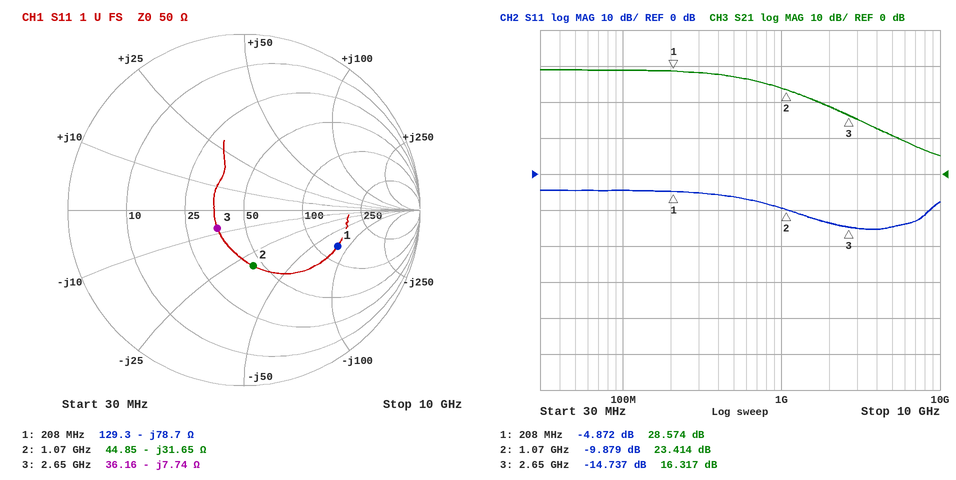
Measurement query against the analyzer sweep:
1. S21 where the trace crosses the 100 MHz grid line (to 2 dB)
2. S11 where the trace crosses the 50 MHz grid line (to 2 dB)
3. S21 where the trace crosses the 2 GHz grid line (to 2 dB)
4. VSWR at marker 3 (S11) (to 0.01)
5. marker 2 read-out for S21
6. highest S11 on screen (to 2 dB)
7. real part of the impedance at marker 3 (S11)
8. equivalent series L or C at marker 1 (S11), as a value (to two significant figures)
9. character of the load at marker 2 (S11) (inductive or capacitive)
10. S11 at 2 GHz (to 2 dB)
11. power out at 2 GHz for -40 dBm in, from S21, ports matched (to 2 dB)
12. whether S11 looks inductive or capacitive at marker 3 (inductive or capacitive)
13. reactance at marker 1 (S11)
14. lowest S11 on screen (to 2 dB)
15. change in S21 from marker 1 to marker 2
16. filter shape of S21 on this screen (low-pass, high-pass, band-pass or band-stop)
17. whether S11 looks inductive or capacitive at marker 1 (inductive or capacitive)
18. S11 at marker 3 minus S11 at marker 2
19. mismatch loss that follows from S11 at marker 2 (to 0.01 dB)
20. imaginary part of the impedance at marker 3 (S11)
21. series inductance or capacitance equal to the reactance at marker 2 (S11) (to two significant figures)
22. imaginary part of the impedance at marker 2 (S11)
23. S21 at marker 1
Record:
28 dB
-4 dB
18 dB
1.45
23.414 dB
-4 dB
36.16 Ω
9.7 pF
capacitive
-14 dB
-22 dBm
capacitive
-78.7 Ω
-16 dB
-5.160 dB
low-pass
capacitive
-4.858 dB
0.47 dB
-7.74 Ω
4.7 pF
-31.65 Ω
28.574 dB
